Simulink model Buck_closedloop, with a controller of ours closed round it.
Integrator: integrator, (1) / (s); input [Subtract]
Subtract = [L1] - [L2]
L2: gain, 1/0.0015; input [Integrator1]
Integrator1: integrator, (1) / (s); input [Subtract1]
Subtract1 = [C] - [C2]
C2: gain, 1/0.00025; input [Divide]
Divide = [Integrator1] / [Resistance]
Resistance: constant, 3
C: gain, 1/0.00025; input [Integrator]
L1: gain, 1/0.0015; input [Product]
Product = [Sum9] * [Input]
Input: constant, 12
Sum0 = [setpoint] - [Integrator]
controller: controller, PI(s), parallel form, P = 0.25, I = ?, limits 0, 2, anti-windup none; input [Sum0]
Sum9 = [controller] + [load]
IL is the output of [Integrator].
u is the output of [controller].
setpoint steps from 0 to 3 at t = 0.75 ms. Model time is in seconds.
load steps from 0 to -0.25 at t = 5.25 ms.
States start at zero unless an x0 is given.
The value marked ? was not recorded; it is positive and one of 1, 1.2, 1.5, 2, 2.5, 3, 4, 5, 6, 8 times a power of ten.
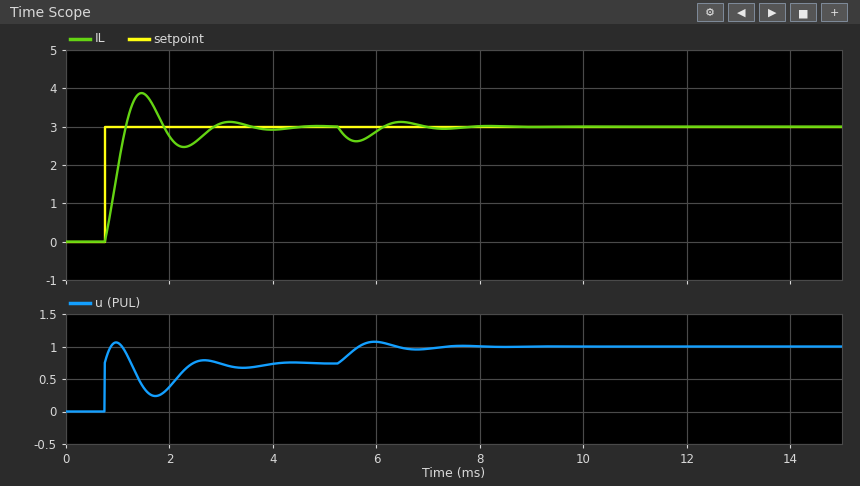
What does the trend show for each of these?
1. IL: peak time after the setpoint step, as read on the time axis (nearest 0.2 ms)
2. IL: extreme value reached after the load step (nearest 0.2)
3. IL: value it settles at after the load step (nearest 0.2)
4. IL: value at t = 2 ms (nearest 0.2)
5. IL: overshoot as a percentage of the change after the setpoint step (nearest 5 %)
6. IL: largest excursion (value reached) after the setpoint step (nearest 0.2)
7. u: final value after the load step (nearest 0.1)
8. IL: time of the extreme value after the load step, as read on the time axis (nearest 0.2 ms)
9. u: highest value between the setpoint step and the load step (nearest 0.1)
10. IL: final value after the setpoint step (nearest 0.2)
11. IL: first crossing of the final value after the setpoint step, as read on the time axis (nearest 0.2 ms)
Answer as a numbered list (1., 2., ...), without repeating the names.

1. 1.4 ms
2. 2.6
3. 3.0
4. 2.8
5. 30 %
6. 3.8
7. 1.0
8. 5.6 ms
9. 1.1
10. 3.0
11. 1.2 ms
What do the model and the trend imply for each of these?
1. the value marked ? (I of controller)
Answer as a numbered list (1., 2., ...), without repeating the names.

1. 1500
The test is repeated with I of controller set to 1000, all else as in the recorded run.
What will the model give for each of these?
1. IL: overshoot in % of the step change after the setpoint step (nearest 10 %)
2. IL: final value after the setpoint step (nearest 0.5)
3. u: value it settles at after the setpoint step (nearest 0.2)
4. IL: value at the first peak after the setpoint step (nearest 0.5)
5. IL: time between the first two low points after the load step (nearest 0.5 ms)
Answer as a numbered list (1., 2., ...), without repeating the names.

1. 20 %
2. 3.0
3. 0.8
4. 3.5
5. 2.0 ms
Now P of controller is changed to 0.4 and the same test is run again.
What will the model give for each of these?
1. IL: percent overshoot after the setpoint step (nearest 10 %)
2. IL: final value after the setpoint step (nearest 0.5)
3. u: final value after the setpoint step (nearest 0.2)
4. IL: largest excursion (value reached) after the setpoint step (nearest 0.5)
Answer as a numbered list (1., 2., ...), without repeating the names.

1. 20 %
2. 3.0
3. 0.8
4. 3.5
